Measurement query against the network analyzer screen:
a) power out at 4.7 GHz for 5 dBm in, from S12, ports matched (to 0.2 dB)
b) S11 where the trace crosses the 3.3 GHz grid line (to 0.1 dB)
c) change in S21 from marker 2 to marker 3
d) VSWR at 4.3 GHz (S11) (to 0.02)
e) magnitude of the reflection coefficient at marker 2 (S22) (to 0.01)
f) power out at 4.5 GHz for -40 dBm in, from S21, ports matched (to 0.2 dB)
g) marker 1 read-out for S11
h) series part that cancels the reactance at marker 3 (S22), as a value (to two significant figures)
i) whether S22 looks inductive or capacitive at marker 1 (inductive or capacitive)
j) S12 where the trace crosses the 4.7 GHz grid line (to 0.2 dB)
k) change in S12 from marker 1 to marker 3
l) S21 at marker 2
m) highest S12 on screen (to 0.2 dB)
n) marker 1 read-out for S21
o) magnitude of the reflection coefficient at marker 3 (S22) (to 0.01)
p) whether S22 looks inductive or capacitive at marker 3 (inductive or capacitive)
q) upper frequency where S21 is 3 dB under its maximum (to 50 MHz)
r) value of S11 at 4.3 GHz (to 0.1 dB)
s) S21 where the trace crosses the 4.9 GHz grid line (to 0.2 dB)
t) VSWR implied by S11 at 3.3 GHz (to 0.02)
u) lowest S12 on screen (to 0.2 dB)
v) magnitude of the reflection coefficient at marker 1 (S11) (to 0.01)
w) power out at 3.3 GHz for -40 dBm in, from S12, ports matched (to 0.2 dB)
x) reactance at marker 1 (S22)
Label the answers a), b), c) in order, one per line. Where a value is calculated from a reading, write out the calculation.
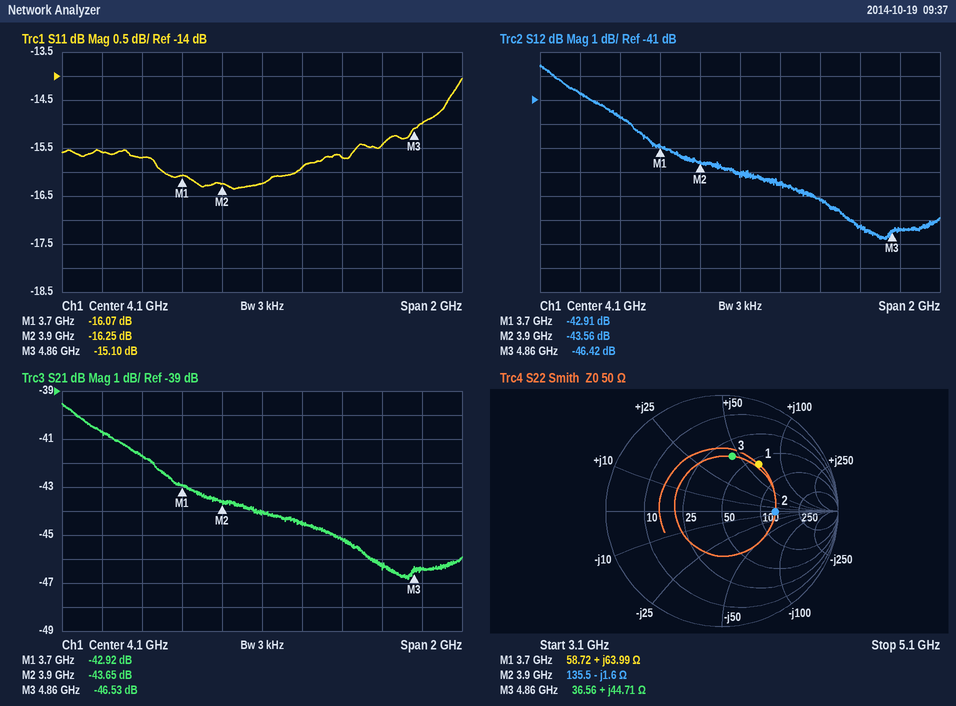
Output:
a) 5 dBm + (-46.2 dB) = -41.2 dBm
b) -15.6 dB
c) -46.53 − (-43.65) = -2.88 dB
d) |Γ| = 10^(-15.9/20) = 0.1603; VSWR = (1 + 0.1603)/(1 − 0.1603) ≈ 1.38
e) 0.46
f) -40 dBm + (-45.2 dB) = -85.2 dBm
g) -16.07 dB
h) C = 1/(2π × 4.86 GHz × 44.71 Ω) ≈ 732 fF, so 730 fF to two significant figures
i) inductive
j) -46.2 dB
k) -46.42 − (-42.91) = -3.51 dB
l) -43.65 dB
m) -39.6 dB
n) -42.92 dB
o) 0.48
p) inductive
q) 3.60 GHz
r) -15.9 dB
s) -46.4 dB
t) |Γ| = 10^(-15.6/20) = 0.1660; VSWR = (1 + 0.1660)/(1 − 0.1660) ≈ 1.40
u) -46.8 dB
v) 10^(-16.07/20) ≈ 0.16
w) -40 dBm + (-40.8 dB) = -80.8 dBm
x) +63.99 Ω
